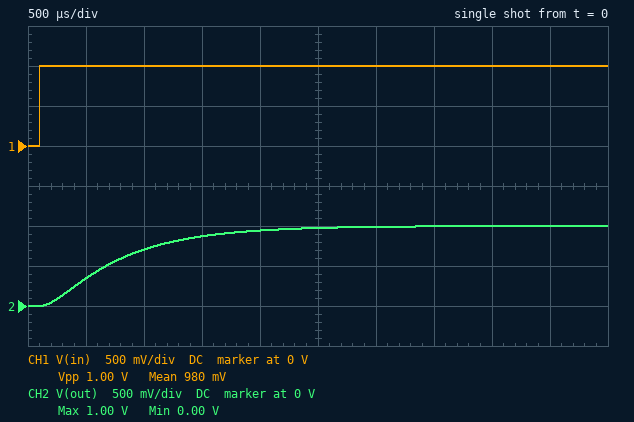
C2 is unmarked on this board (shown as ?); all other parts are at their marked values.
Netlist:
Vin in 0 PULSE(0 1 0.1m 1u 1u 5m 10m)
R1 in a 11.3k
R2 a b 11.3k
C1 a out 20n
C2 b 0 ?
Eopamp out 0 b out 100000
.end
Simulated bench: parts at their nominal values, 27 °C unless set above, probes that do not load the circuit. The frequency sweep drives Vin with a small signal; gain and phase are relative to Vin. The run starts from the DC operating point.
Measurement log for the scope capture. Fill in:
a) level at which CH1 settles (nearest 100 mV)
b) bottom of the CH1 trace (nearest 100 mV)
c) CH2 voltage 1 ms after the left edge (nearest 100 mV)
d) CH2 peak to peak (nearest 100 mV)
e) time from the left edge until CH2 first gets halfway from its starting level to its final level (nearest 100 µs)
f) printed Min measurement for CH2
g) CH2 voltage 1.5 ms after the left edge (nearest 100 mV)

1.0 V
0 V
700 mV
1.0 V
700 µs
0.00 V
900 mV
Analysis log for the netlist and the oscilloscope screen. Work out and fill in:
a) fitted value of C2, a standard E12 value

33 nF
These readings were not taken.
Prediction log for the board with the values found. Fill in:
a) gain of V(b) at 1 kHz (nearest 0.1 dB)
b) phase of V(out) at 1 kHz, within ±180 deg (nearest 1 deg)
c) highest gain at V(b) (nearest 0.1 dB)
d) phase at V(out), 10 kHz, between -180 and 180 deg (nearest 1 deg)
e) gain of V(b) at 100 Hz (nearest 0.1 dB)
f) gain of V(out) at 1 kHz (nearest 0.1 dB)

-14.4 dB
-116 deg
0 dB
-172 deg
-0.6 dB
-14.4 dB
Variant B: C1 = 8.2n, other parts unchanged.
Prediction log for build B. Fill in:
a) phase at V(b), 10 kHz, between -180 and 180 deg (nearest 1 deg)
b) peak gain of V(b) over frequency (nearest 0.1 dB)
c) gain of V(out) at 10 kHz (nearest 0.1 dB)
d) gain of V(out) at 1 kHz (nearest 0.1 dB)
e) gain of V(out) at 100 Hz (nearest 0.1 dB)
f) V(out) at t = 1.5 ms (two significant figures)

-161 deg
0 dB
-43.1 dB
-13.4 dB
-0.8 dB
860 mV
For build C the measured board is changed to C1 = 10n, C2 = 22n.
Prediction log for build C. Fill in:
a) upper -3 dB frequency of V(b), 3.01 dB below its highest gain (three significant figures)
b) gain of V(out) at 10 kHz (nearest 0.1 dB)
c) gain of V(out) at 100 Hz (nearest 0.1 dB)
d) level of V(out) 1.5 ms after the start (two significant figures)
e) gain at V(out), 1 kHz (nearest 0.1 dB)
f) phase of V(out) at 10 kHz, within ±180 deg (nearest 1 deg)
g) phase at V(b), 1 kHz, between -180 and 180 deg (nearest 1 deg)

360 Hz
-41.2 dB
-0.3 dB
950 mV
-9.9 dB
-164 deg
-92 deg
